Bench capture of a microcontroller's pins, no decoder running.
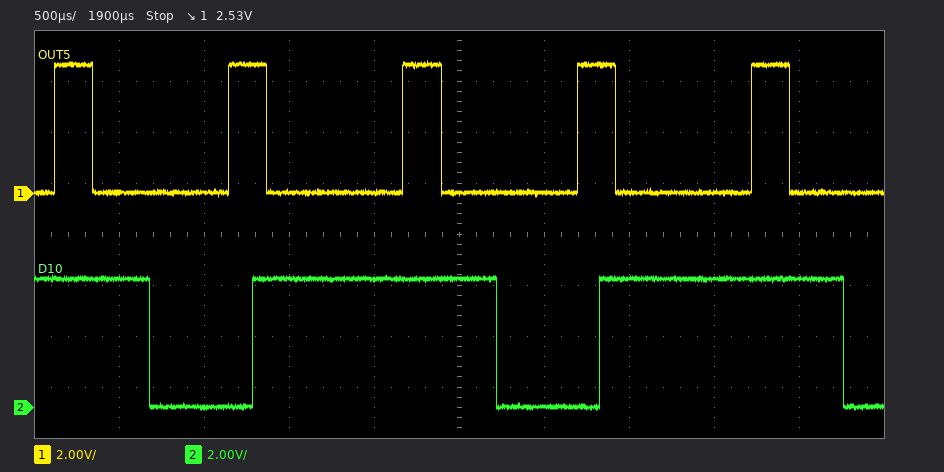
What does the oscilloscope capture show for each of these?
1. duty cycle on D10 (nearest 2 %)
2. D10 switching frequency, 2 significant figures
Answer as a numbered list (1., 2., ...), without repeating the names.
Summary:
1. 70 %
2. 490 Hz
